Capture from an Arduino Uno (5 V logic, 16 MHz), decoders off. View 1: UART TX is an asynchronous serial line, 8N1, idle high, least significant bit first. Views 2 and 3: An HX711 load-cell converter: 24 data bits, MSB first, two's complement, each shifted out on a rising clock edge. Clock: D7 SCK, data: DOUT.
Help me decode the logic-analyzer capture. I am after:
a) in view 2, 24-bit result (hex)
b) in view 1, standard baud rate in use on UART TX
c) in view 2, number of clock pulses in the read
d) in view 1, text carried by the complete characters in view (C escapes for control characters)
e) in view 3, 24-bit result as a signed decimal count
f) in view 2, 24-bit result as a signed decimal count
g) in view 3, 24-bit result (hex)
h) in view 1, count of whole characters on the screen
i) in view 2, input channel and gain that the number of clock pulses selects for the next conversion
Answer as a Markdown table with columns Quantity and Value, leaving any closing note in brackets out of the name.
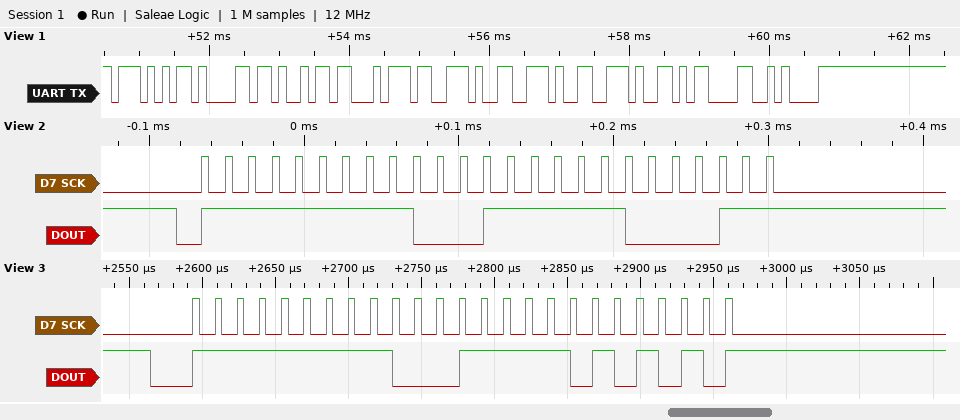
| Quantity | Value |
|---|---|
| in view 2, 24-bit result | 0xFF8FC3 |
| in view 1, standard baud rate in use on UART TX | 9600 baud |
| in view 2, number of clock pulses in the read | 25 |
| in view 1, text carried by the complete characters in view | "Wait...\r\n" |
| in view 3, 24-bit result as a signed decimal count | -28758 |
| in view 2, 24-bit result as a signed decimal count | -28733 |
| in view 3, 24-bit result | 0xFF8FAA |
| in view 1, count of whole characters on the screen | 9 |
| in view 2, input channel and gain that the number of clock pulses selects for the next conversion | channel A, gain 128 |
